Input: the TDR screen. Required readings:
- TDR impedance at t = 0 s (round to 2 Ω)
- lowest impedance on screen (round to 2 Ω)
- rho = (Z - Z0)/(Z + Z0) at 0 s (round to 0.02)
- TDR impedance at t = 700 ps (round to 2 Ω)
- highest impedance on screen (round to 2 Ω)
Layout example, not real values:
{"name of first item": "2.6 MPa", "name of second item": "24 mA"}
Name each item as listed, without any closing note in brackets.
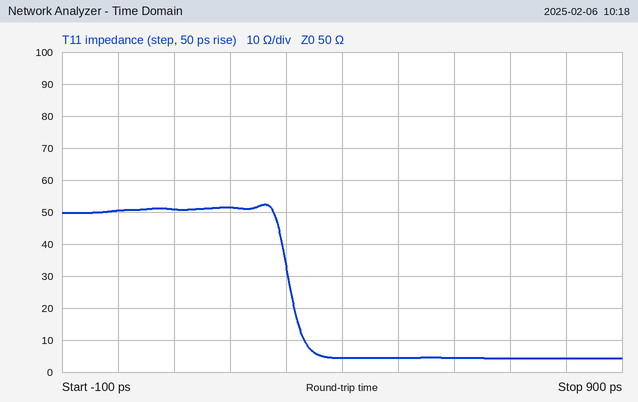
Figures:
{"TDR impedance at t = 0 s": "50 Ω", "lowest impedance on screen": "4 Ω", "rho = (Z - Z0)/(Z + Z0) at 0 s": "0.00", "TDR impedance at t = 700 ps": "4 Ω", "highest impedance on screen": "52 Ω"}
